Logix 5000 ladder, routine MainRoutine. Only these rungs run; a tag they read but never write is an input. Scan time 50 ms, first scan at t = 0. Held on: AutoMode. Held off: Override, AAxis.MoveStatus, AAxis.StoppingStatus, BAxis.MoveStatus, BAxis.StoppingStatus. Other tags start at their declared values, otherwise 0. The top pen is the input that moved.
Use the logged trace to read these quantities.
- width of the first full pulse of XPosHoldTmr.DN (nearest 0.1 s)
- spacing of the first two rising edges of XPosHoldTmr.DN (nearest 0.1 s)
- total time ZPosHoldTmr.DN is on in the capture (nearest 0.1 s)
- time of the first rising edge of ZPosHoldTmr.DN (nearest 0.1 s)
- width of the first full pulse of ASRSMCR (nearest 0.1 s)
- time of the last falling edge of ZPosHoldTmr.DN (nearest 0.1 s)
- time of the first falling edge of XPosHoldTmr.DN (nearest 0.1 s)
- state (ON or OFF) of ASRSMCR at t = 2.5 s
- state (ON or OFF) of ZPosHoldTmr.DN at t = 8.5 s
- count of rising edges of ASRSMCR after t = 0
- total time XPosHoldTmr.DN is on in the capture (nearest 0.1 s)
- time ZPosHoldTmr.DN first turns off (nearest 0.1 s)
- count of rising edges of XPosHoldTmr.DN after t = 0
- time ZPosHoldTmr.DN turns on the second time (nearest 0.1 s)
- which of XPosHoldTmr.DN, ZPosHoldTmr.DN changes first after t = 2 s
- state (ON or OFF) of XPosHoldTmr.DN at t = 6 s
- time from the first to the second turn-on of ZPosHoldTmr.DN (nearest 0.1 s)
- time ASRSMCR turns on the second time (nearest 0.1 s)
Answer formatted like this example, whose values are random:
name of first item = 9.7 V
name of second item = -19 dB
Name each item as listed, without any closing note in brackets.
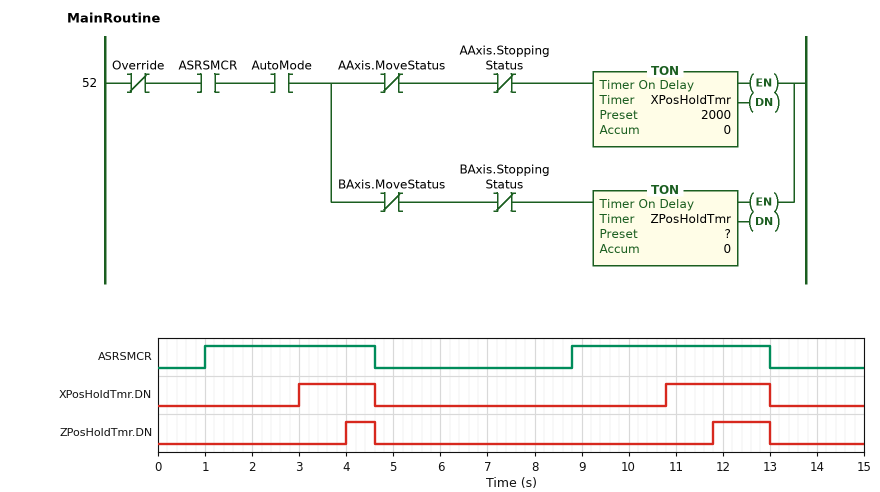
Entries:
width of the first full pulse of XPosHoldTmr.DN = 1.6 s
spacing of the first two rising edges of XPosHoldTmr.DN = 7.8 s
total time ZPosHoldTmr.DN is on in the capture = 1.8 s
time of the first rising edge of ZPosHoldTmr.DN = 4.0 s
width of the first full pulse of ASRSMCR = 3.6 s
time of the last falling edge of ZPosHoldTmr.DN = 13.0 s
time of the first falling edge of XPosHoldTmr.DN = 4.6 s
state (ON or OFF) of ASRSMCR at t = 2.5 s = ON
state (ON or OFF) of ZPosHoldTmr.DN at t = 8.5 s = OFF
count of rising edges of ASRSMCR after t = 0 = 2
total time XPosHoldTmr.DN is on in the capture = 3.8 s
time ZPosHoldTmr.DN first turns off = 4.6 s
count of rising edges of XPosHoldTmr.DN after t = 0 = 2
time ZPosHoldTmr.DN turns on the second time = 11.8 s
which of XPosHoldTmr.DN, ZPosHoldTmr.DN changes first after t = 2 s = XPosHoldTmr.DN
state (ON or OFF) of XPosHoldTmr.DN at t = 6 s = OFF
time from the first to the second turn-on of ZPosHoldTmr.DN = 7.8 s
time ASRSMCR turns on the second time = 8.8 s
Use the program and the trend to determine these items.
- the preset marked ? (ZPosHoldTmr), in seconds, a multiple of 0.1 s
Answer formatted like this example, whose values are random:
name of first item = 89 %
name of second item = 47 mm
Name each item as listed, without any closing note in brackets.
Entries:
the preset marked ? (ZPosHoldTmr), in seconds, a multiple of 0.1 s = 3.0 s
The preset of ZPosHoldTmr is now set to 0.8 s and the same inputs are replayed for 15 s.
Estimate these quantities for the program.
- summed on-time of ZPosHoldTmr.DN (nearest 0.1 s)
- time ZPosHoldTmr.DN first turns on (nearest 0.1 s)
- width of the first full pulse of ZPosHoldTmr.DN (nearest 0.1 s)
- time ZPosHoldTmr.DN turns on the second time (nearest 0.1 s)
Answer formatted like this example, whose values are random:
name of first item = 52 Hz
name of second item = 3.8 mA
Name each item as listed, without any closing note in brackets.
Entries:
summed on-time of ZPosHoldTmr.DN = 6.2 s
time ZPosHoldTmr.DN first turns on = 1.8 s
width of the first full pulse of ZPosHoldTmr.DN = 2.8 s
time ZPosHoldTmr.DN turns on the second time = 9.6 s
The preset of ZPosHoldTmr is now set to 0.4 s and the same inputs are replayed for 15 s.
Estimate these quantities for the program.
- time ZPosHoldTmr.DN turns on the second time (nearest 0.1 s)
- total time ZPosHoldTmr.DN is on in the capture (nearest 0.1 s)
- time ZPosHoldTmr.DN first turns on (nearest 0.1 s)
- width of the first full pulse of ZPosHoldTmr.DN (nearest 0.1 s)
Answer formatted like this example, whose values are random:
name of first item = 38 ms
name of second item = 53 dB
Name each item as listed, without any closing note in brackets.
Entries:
time ZPosHoldTmr.DN turns on the second time = 9.2 s
total time ZPosHoldTmr.DN is on in the capture = 7.0 s
time ZPosHoldTmr.DN first turns on = 1.4 s
width of the first full pulse of ZPosHoldTmr.DN = 3.2 s
